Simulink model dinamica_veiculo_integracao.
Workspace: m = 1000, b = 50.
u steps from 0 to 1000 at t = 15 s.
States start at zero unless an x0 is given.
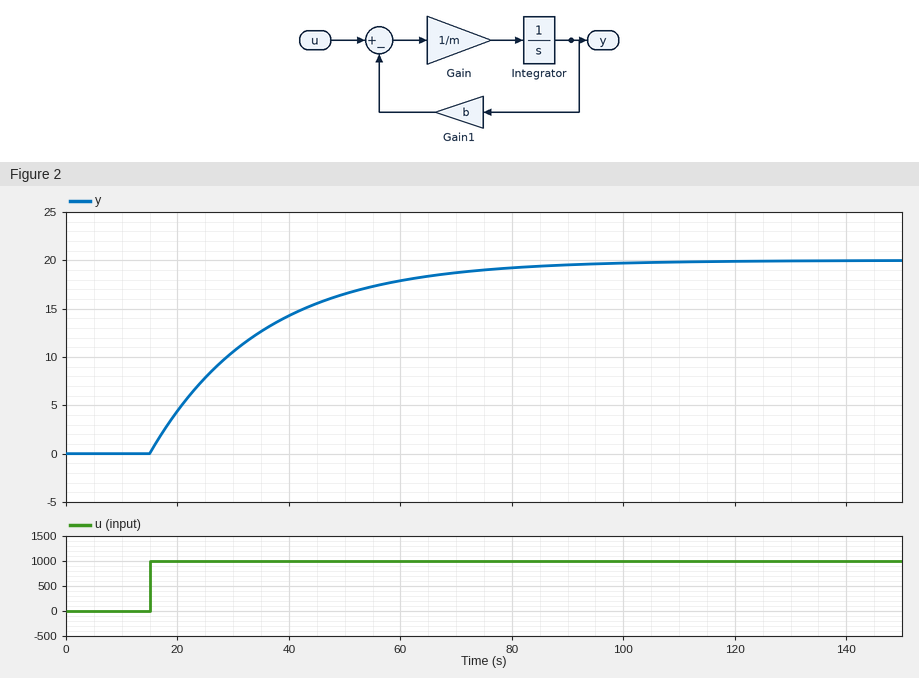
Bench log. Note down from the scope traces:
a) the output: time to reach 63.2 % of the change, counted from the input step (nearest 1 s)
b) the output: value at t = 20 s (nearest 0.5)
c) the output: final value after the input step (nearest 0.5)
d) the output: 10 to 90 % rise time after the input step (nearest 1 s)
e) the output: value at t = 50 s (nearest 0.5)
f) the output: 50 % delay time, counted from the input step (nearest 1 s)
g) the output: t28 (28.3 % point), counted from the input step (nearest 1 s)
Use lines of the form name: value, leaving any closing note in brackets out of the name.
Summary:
the output: time to reach 63.2 % of the change, counted from the input step: 20 s
the output: value at t = 20 s: 4.5
the output: final value after the input step: 20.0
the output: 10 to 90 % rise time after the input step: 44 s
the output: value at t = 50 s: 16.5
the output: 50 % delay time, counted from the input step: 14 s
the output: t28 (28.3 % point), counted from the input step: 7 s
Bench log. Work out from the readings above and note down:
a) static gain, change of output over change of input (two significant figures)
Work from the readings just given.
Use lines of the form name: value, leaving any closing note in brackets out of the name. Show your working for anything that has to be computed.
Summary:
static gain, change of output over change of input: (20 - 0) / (1000 - 0) = 0.020
